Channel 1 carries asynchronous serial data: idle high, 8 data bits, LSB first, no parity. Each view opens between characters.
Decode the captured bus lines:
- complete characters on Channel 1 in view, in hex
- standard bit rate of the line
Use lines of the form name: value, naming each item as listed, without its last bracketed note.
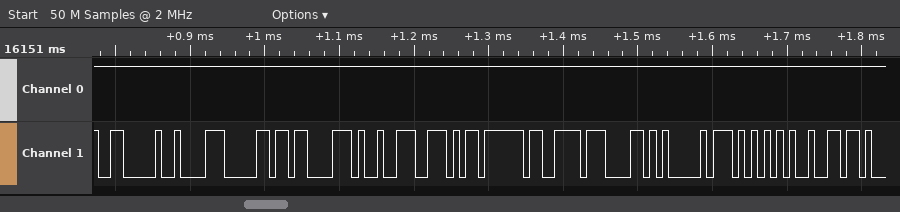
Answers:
complete characters on Channel 1 in view, in hex: 06, C2, B0, C3, C9, AE, BF, DE, 58, D0, 55, B2
standard bit rate of the line: 115200 baud
